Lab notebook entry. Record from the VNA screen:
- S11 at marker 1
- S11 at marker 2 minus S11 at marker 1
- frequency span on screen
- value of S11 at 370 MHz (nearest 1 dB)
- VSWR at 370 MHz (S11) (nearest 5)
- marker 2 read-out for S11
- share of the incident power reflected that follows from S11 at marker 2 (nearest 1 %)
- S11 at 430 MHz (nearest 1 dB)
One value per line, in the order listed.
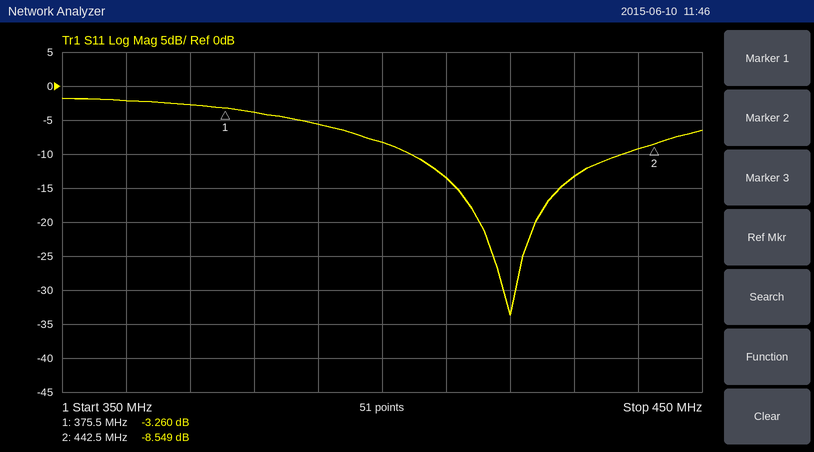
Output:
-3.260 dB
-5.289 dB
100 MHz
-3 dB
5
-8.549 dB
14 %
-13 dB
